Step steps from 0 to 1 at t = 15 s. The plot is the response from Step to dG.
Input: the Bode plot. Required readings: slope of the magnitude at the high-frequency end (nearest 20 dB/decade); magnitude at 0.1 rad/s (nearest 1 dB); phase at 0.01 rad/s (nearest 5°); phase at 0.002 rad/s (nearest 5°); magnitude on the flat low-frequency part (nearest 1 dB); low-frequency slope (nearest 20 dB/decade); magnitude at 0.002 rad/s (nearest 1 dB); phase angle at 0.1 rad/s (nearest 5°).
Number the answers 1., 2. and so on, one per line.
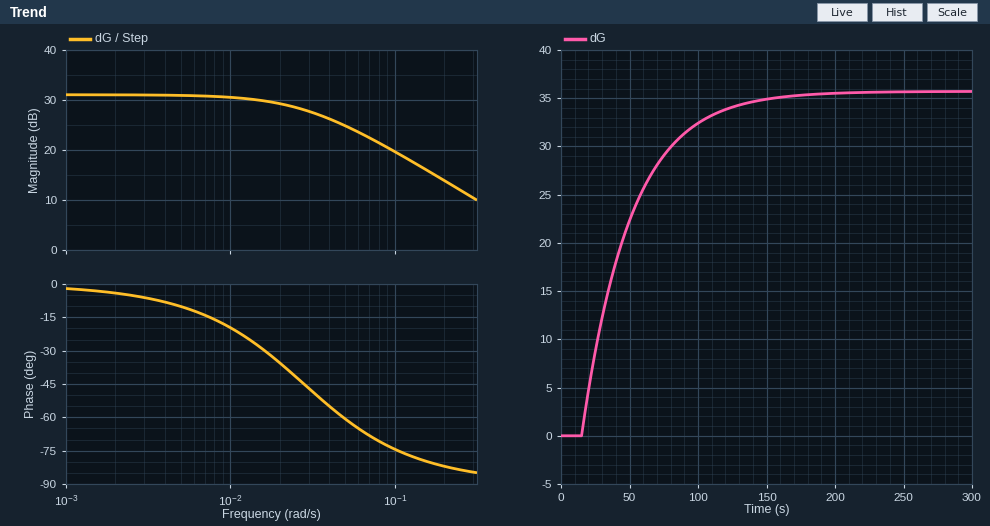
1. -20 dB/decade
2. 20 dB
3. -20°
4. -5°
5. 31 dB
6. 0 dB/decade
7. 31 dB
8. -75°
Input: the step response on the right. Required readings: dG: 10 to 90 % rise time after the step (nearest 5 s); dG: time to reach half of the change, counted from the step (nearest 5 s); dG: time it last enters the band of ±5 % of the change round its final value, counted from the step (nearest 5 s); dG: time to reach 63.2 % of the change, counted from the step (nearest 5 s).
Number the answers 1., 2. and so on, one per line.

1. 80 s
2. 25 s
3. 105 s
4. 35 s
